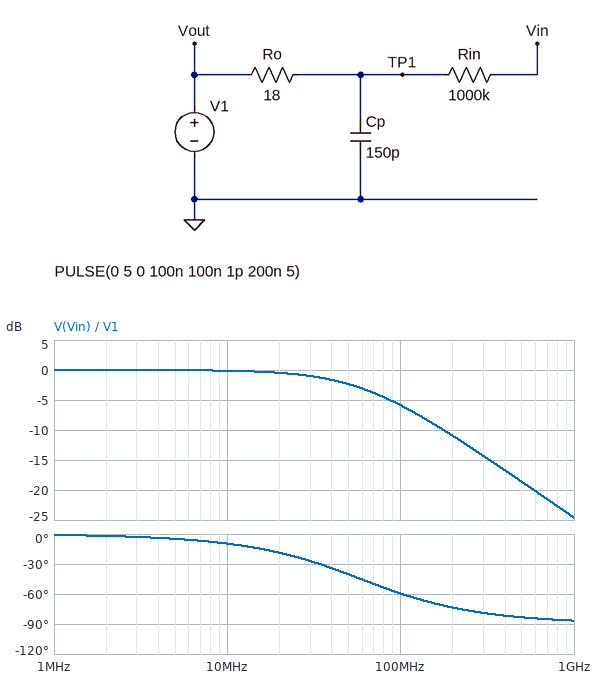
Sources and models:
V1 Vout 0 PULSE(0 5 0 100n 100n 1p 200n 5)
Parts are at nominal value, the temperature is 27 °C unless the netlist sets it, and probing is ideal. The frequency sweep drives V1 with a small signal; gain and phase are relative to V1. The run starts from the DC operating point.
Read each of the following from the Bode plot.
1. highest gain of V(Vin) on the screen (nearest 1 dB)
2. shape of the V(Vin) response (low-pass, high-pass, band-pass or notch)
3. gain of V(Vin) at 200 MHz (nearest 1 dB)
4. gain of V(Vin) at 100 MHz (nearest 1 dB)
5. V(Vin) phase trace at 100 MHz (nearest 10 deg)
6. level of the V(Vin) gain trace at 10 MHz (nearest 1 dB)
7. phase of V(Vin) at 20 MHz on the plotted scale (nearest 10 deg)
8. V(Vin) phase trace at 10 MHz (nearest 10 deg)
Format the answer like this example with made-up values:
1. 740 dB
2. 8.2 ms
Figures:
1. 0 dB
2. low-pass
3. -11 dB
4. -6 dB
5. -60 deg
6. 0 dB
7. -20 deg
8. -10 deg
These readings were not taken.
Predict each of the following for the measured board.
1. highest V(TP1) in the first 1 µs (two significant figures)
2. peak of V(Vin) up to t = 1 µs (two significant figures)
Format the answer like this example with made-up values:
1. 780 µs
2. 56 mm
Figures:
1. 4.9 V
2. 4.9 V
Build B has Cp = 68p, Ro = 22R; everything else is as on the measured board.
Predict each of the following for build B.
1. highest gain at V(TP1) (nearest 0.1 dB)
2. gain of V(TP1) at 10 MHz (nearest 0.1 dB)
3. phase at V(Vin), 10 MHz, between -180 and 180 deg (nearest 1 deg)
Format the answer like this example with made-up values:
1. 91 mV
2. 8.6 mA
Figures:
1. 0 dB
2. 0 dB
3. -5 deg
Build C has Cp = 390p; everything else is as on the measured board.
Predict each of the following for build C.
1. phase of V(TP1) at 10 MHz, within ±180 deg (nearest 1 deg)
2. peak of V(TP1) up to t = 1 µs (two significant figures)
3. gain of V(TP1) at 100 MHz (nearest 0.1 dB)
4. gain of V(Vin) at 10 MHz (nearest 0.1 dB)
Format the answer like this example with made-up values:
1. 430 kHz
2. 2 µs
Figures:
1. -24 deg
2. 4.8 V
3. -13.1 dB
4. -0.8 dB
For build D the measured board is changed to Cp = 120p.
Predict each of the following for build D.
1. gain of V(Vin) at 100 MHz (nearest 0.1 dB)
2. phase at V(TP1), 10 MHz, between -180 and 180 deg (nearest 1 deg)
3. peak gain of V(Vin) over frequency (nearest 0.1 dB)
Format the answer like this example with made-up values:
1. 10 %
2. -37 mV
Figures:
1. -4.5 dB
2. -8 deg
3. 0 dB
